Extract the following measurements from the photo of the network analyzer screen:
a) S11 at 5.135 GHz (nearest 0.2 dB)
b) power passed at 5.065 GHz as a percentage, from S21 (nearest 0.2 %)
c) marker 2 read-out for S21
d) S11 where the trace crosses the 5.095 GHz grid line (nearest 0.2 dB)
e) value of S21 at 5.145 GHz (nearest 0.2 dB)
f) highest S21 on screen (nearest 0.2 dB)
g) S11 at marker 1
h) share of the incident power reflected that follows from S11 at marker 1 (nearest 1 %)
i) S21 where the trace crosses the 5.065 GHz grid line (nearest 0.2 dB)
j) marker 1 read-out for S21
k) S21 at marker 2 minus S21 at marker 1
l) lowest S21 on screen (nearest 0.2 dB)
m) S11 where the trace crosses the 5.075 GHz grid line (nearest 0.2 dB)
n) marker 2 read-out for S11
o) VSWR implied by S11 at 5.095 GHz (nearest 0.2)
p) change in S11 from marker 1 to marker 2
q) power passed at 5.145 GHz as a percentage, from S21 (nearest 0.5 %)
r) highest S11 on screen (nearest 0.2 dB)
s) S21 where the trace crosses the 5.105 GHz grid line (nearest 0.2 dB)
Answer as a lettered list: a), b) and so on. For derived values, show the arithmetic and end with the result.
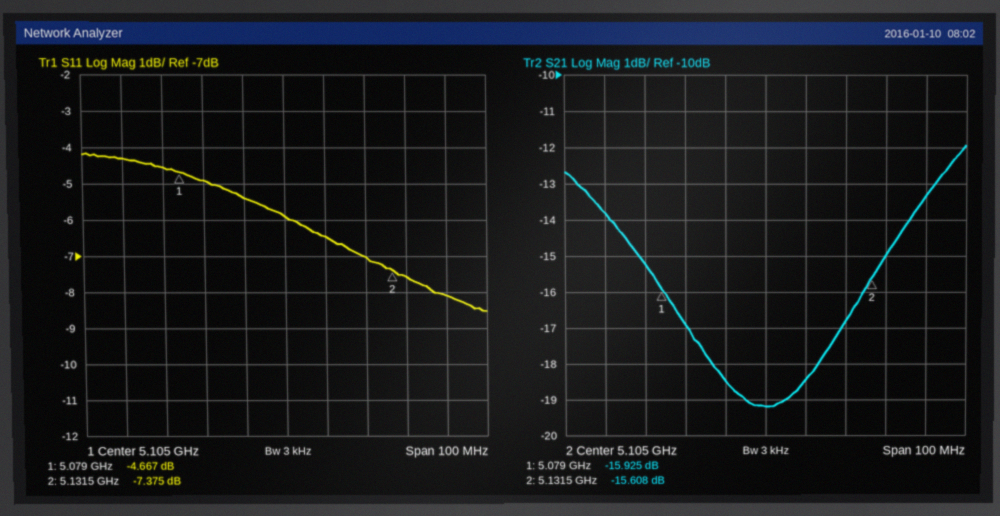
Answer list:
a) -7.6 dB
b) 10^(-13.8/10) ≈ 4.2 %
c) -15.608 dB
d) -5.4 dB
e) -13.4 dB
f) -12.0 dB
g) -4.667 dB
h) 10^(-4.667/10) ≈ 34 %
i) -13.8 dB
j) -15.925 dB
k) -15.608 − (-15.925) = 0.317 dB
l) -19.2 dB
m) -4.6 dB
n) -7.375 dB
o) |Γ| = 10^(-5.4/20) = 0.5370; VSWR = (1 + 0.5370)/(1 − 0.5370) ≈ 3.32, so 3.4 to the nearest 0.2
p) -7.375 − (-4.667) = -2.708 dB
q) 10^(-13.4/10) ≈ 4.57 %, so 4.5 % to the nearest 0.5 %
r) -4.2 dB
s) -19.2 dB
